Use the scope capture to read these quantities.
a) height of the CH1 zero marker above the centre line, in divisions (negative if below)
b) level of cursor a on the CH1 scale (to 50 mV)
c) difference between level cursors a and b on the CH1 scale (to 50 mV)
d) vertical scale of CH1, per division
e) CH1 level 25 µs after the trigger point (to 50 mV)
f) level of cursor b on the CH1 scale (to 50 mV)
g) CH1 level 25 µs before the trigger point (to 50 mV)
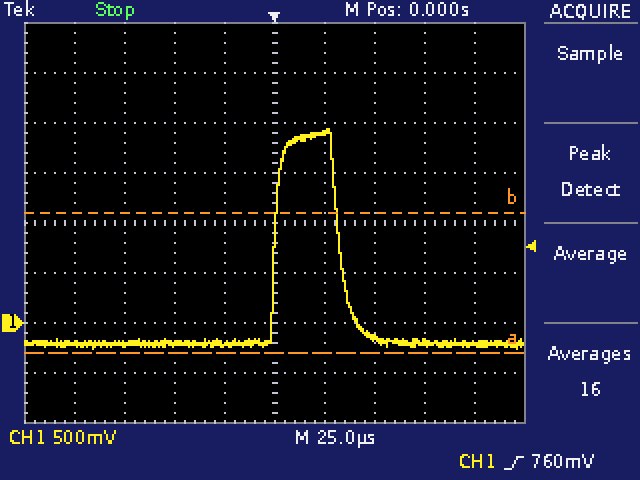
-2.0 div
-300 mV
1.40 V
500 mV
1.90 V
1.10 V
-200 mV
